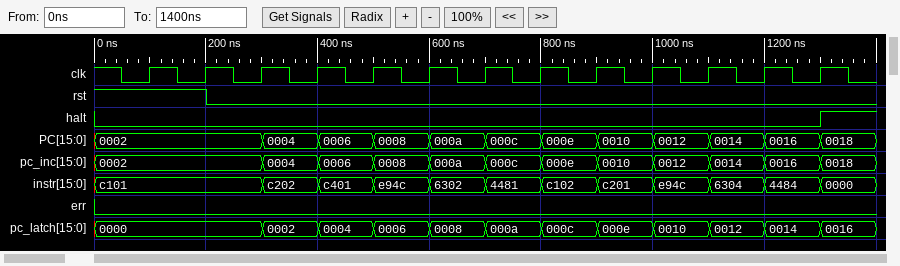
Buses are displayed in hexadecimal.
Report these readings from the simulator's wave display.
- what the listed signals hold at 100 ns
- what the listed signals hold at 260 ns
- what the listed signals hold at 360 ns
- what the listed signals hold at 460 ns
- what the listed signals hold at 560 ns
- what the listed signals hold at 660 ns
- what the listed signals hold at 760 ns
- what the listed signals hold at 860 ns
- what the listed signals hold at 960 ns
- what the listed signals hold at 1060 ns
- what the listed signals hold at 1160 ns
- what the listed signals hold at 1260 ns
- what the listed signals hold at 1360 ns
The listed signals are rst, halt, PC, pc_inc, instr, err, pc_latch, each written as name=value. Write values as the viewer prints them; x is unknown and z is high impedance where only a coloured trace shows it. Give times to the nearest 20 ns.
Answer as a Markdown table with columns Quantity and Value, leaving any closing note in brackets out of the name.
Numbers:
| Quantity | Value |
|---|---|
| what the listed signals hold at 100 ns | rst=1, halt=0, PC=0002, pc_inc=0002, instr=c101, err=0, pc_latch=0000 |
| what the listed signals hold at 260 ns | rst=0, halt=0, PC=0002, pc_inc=0002, instr=c101, err=0, pc_latch=0000 |
| what the listed signals hold at 360 ns | rst=0, halt=0, PC=0004, pc_inc=0004, instr=c202, err=0, pc_latch=0002 |
| what the listed signals hold at 460 ns | rst=0, halt=0, PC=0006, pc_inc=0006, instr=c401, err=0, pc_latch=0004 |
| what the listed signals hold at 560 ns | rst=0, halt=0, PC=0008, pc_inc=0008, instr=e94c, err=0, pc_latch=0006 |
| what the listed signals hold at 660 ns | rst=0, halt=0, PC=000a, pc_inc=000a, instr=6302, err=0, pc_latch=0008 |
| what the listed signals hold at 760 ns | rst=0, halt=0, PC=000c, pc_inc=000c, instr=4481, err=0, pc_latch=000a |
| what the listed signals hold at 860 ns | rst=0, halt=0, PC=000e, pc_inc=000e, instr=c102, err=0, pc_latch=000c |
| what the listed signals hold at 960 ns | rst=0, halt=0, PC=0010, pc_inc=0010, instr=c201, err=0, pc_latch=000e |
| what the listed signals hold at 1060 ns | rst=0, halt=0, PC=0012, pc_inc=0012, instr=e94c, err=0, pc_latch=0010 |
| what the listed signals hold at 1160 ns | rst=0, halt=0, PC=0014, pc_inc=0014, instr=6304, err=0, pc_latch=0012 |
| what the listed signals hold at 1260 ns | rst=0, halt=0, PC=0016, pc_inc=0016, instr=4484, err=0, pc_latch=0014 |
| what the listed signals hold at 1360 ns | rst=0, halt=1, PC=0018, pc_inc=0018, instr=0000, err=0, pc_latch=0016 |
